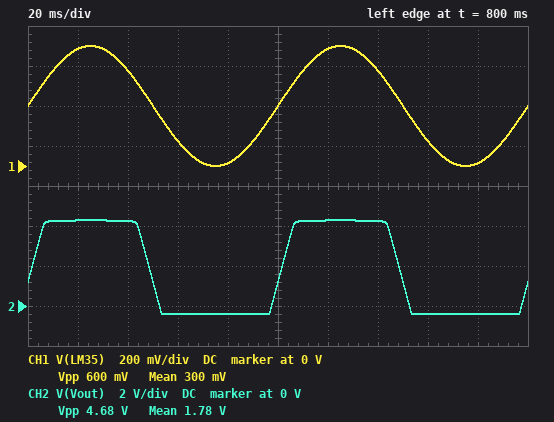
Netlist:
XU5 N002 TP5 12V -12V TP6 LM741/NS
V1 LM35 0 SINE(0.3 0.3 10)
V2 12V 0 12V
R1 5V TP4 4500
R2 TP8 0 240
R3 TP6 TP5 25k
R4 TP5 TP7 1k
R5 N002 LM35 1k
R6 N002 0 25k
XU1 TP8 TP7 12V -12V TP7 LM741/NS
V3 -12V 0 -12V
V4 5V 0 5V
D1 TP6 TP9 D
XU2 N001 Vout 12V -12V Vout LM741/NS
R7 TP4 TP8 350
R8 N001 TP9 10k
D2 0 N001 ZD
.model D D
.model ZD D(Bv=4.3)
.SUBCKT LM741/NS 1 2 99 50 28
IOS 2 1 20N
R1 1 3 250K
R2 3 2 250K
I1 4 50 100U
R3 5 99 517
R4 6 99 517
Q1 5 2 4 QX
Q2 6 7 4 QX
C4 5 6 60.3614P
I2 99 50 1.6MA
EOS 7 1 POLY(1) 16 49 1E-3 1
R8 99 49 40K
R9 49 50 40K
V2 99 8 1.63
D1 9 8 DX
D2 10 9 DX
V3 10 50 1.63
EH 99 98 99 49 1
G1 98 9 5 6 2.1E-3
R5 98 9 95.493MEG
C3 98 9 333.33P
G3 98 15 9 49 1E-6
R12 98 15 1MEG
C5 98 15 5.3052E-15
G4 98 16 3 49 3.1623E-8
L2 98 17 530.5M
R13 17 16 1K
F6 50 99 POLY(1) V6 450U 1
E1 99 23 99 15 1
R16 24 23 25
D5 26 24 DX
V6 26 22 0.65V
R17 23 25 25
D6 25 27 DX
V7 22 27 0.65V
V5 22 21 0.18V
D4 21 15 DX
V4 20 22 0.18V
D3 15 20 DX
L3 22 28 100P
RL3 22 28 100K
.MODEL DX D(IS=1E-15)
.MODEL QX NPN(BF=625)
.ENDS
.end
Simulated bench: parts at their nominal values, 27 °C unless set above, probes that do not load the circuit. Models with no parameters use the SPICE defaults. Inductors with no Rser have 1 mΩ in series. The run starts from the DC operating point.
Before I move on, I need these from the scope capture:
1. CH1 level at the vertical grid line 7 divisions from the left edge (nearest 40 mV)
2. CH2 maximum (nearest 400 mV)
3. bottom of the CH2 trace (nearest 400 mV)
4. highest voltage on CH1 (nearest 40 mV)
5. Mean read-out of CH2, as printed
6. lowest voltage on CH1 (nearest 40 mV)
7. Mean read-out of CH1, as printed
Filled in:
480 mV
4.4 V
-400 mV
600 mV
1.78 V
0 V
300 mV
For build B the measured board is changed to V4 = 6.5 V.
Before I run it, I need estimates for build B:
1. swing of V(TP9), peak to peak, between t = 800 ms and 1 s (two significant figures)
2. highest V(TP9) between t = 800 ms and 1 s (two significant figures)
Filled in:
7.1 V
6.7 V
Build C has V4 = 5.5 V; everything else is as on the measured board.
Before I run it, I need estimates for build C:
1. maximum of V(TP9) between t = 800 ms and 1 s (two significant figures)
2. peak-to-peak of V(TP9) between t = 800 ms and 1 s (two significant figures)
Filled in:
7.9 V
8.3 V
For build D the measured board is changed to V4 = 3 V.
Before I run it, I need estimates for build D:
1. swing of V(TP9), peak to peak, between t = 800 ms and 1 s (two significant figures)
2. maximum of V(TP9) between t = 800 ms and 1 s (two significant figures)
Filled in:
11 V
10 V
